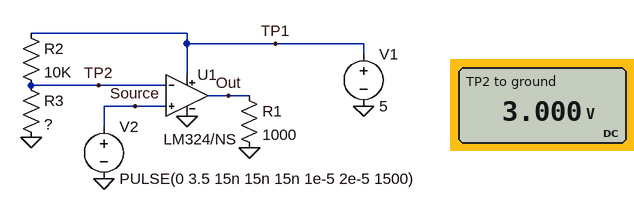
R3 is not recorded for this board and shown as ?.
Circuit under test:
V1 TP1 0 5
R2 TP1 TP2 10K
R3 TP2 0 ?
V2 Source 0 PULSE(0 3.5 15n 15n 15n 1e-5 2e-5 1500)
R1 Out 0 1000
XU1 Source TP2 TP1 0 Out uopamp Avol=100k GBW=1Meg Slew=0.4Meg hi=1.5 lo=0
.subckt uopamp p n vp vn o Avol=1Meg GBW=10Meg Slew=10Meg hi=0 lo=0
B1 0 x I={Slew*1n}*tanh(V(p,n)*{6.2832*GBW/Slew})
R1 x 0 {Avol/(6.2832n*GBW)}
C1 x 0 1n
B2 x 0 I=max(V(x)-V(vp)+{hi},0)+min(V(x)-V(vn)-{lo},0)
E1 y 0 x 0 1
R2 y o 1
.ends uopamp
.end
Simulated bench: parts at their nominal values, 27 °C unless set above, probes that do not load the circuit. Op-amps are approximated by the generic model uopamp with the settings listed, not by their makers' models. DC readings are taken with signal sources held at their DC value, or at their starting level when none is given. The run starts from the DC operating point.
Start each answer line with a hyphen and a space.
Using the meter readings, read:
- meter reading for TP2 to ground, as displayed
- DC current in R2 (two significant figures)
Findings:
- 3.000 V
- 200 µA
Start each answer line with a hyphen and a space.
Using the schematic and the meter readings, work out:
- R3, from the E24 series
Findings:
- 15 kΩ
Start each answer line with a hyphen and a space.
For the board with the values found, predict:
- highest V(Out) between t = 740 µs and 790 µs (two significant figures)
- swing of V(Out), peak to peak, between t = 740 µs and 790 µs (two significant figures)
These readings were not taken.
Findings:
- 3.5 V
- 3.5 V
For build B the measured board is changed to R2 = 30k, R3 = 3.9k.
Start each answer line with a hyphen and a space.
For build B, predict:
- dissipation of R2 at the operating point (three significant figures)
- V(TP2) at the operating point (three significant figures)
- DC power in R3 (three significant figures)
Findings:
- 653 µW
- 575 mV
- 84.8 µW
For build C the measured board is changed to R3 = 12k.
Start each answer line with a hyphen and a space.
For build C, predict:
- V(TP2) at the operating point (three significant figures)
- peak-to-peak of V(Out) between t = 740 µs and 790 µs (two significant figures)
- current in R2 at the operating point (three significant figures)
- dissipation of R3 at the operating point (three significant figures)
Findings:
- 2.73 V
- 3.5 V
- 227 µA
- 620 µW
